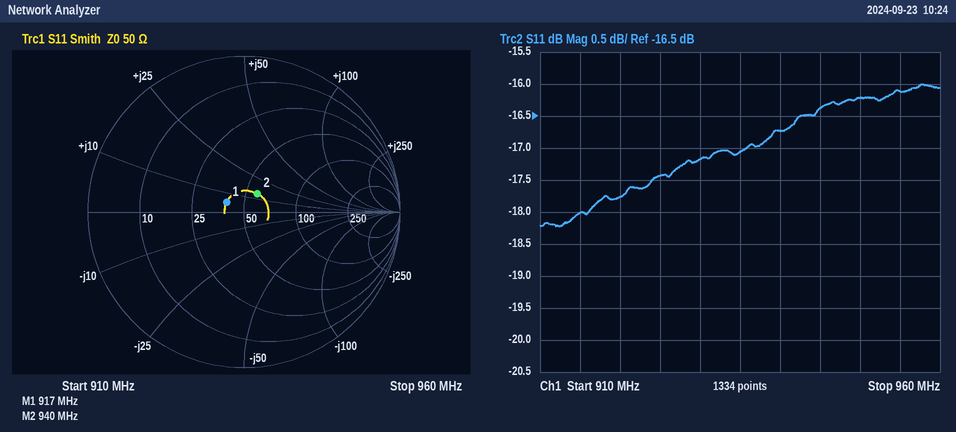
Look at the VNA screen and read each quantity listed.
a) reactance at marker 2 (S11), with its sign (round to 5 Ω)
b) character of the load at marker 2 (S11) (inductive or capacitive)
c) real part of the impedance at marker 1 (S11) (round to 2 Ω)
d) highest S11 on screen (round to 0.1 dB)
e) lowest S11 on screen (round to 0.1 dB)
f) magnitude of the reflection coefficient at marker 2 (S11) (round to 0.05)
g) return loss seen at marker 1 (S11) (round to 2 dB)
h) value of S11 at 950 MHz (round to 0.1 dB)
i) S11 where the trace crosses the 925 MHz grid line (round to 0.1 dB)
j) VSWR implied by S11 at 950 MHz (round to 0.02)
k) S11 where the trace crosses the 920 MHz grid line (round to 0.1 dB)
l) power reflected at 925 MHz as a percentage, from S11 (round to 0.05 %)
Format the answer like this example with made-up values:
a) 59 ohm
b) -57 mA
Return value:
a) +15 Ω
b) inductive
c) 40 Ω
d) -16.0 dB
e) -18.2 dB
f) 0.15
g) 18 dB
h) -16.2 dB
i) -17.4 dB
j) 1.36
k) -17.8 dB
l) 1.80 %
